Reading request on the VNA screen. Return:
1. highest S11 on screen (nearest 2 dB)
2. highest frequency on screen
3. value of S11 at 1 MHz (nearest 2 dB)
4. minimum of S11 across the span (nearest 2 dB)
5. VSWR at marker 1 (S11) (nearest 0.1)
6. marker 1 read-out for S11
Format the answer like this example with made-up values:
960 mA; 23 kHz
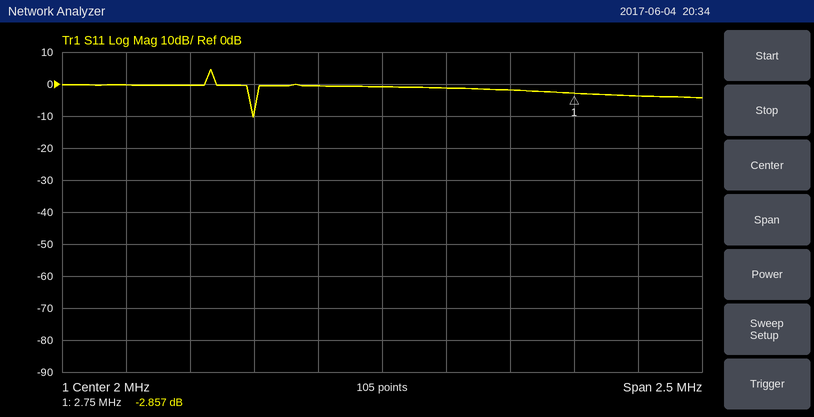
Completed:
4 dB; 3.25 MHz; 0 dB; -10 dB; 6.1; -2.857 dB
